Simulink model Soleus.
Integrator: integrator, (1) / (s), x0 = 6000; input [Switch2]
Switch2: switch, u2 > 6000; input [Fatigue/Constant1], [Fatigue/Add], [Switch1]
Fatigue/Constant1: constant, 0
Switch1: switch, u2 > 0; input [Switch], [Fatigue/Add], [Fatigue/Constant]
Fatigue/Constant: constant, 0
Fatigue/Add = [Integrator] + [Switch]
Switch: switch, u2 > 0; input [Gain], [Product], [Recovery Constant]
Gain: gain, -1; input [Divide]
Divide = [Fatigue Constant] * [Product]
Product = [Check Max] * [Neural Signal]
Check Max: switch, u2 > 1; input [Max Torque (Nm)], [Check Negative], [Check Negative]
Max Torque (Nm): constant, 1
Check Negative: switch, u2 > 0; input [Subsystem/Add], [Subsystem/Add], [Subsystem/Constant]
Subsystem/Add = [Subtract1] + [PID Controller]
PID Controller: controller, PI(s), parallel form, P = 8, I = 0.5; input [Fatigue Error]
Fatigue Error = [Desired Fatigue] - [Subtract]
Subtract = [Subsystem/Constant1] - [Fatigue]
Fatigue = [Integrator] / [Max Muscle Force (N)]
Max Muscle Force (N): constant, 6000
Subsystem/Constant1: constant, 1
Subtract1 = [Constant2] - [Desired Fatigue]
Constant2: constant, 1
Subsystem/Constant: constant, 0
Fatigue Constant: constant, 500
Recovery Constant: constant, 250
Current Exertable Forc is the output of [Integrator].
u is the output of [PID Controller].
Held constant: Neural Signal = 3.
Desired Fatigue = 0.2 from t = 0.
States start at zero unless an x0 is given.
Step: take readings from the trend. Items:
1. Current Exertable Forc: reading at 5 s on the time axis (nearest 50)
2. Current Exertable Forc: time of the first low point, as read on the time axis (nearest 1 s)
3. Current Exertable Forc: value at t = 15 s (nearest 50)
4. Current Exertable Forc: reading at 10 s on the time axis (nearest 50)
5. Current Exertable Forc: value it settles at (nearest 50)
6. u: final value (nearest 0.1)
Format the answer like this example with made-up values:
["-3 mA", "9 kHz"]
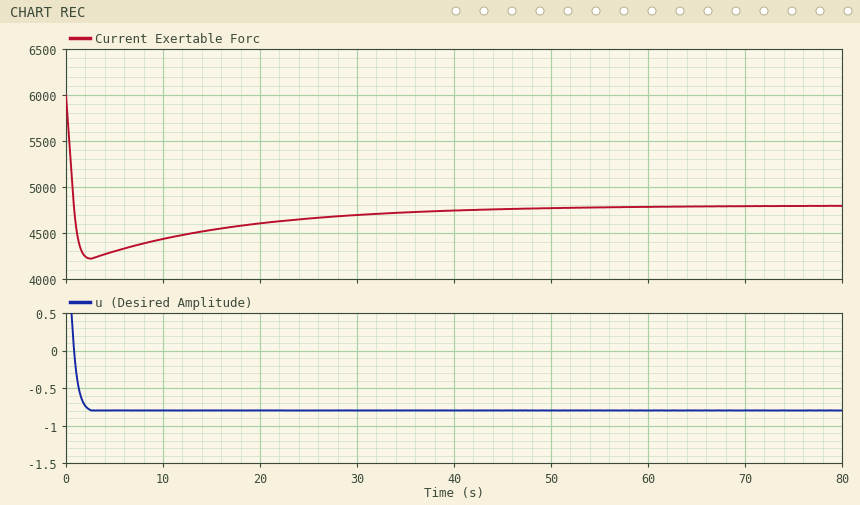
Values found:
["4300", "3 s", "4550", "4450", "4800", "-0.8"]
